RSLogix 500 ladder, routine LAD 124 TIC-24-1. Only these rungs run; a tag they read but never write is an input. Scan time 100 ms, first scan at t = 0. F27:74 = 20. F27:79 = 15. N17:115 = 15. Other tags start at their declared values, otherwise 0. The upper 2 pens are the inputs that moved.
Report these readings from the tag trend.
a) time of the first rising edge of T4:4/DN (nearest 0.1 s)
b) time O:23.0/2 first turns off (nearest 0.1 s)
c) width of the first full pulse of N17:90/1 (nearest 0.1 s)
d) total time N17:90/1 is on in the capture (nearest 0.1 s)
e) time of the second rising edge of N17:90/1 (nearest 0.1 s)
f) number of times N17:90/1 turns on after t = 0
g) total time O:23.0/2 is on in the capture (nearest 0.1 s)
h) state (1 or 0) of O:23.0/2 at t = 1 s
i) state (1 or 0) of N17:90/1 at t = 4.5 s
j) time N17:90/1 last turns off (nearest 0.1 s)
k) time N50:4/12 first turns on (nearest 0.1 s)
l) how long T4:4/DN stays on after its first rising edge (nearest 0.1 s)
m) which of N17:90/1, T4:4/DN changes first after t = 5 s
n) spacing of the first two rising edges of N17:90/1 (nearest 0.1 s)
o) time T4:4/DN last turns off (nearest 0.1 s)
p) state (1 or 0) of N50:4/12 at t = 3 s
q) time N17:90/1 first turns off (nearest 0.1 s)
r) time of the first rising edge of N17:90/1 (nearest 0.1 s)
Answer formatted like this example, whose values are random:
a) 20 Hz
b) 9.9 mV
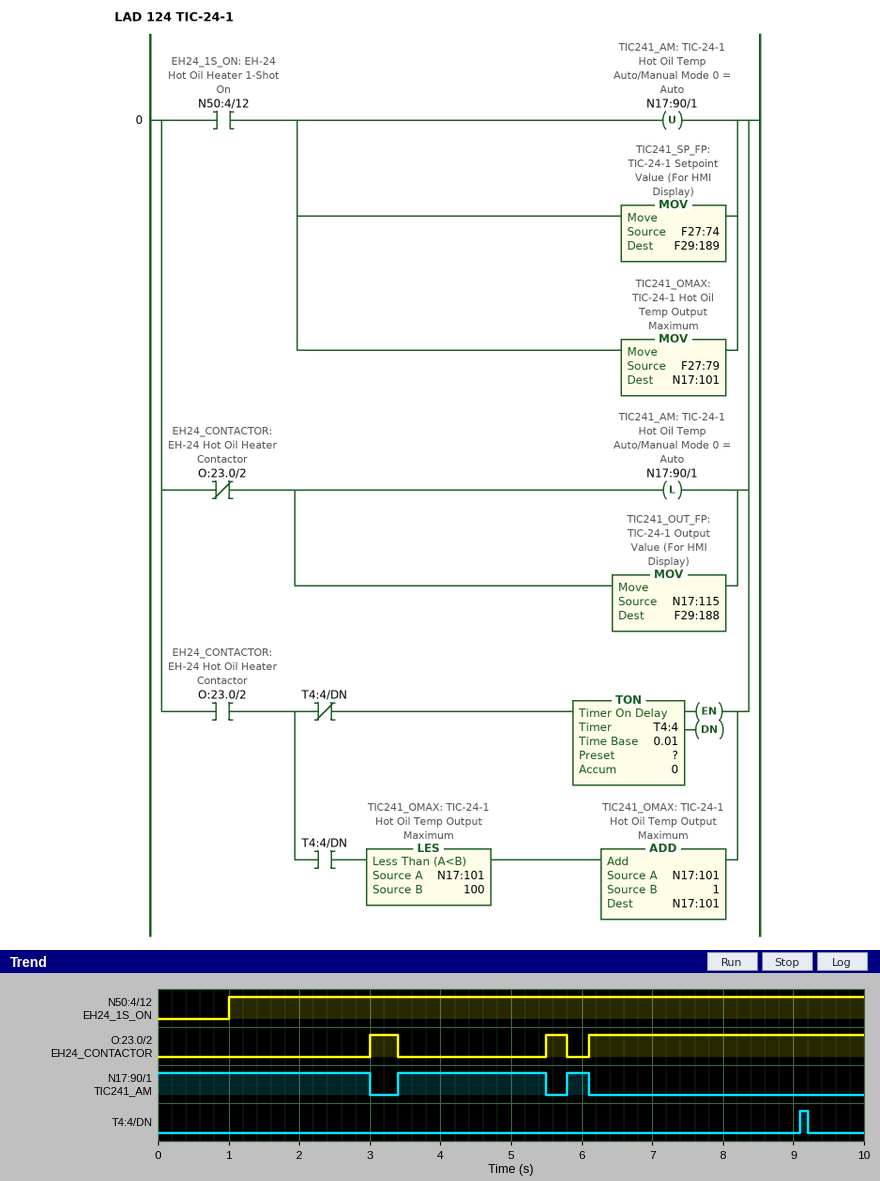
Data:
a) 9.1 s
b) 3.4 s
c) 2.1 s
d) 5.4 s
e) 5.8 s
f) 2
g) 4.6 s
h) 0
i) 1
j) 6.1 s
k) 1.0 s
l) 0.1 s
m) N17:90/1
n) 2.4 s
o) 9.2 s
p) 1
q) 3.0 s
r) 3.4 s
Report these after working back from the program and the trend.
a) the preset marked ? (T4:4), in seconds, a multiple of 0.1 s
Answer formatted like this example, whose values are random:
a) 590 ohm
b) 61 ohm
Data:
a) 3.0 s
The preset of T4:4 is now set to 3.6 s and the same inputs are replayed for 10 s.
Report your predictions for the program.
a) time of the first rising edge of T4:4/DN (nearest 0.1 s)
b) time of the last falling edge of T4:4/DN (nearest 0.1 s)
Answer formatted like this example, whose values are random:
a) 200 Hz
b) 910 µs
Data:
a) 9.7 s
b) 9.8 s
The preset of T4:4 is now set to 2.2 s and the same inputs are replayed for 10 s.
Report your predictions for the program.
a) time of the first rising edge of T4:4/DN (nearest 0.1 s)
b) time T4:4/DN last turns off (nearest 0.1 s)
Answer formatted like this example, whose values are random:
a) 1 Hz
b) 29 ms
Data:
a) 8.3 s
b) 8.4 s
